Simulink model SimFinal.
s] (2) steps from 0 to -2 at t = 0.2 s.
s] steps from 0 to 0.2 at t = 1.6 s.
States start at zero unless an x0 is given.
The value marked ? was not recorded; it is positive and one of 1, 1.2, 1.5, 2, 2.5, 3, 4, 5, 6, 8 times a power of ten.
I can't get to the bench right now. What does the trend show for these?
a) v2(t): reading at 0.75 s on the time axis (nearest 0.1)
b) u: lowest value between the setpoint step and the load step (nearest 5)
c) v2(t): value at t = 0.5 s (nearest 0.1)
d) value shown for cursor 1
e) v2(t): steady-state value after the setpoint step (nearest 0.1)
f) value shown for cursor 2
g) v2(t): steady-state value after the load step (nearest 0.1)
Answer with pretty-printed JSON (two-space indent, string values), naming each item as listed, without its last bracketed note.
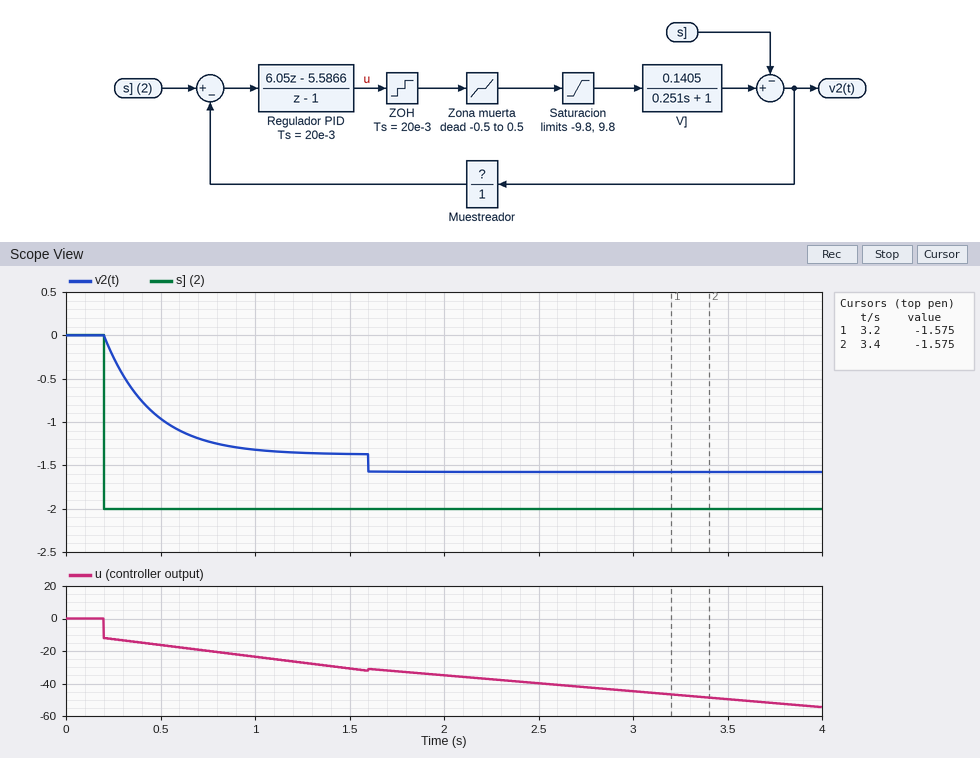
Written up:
{
  "v2(t): reading at 0.75 s on the time axis": "-1.2",
  "u: lowest value between the setpoint step and the load step": "-30",
  "v2(t): value at t = 0.5 s": "-1.0",
  "value shown for cursor 1": "-1.575",
  "v2(t): steady-state value after the setpoint step": "-1.4",
  "value shown for cursor 2": "-1.575",
  "v2(t): steady-state value after the load step": "-1.6"
}
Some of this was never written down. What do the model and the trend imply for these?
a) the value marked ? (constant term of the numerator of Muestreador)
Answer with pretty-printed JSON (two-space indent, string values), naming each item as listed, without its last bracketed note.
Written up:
{
  "the value marked ?": "1"
}
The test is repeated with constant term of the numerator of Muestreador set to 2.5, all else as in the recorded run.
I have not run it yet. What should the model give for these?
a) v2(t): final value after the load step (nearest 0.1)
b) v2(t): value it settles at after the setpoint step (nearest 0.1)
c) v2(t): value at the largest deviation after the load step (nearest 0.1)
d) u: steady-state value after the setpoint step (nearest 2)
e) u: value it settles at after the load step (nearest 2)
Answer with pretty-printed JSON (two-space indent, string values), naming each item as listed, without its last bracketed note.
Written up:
{
  "v2(t): final value after the load step": "-0.8",
  "v2(t): value it settles at after the setpoint step": "-0.8",
  "v2(t): value at the largest deviation after the load step": "-1.0",
  "u: steady-state value after the setpoint step": "-6",
  "u: value it settles at after the load step": "-4"
}
